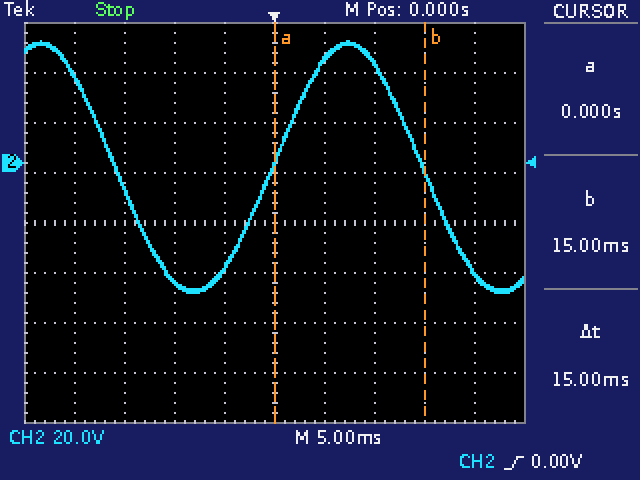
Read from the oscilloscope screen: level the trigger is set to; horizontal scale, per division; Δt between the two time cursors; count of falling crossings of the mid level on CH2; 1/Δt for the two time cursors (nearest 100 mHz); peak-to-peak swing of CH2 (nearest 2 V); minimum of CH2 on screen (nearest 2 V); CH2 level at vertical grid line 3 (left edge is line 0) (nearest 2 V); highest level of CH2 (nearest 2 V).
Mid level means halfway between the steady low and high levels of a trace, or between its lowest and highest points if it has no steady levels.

0.00 V
5 ms
15 ms
2
66.7 Hz
100 V
-52 V
-48 V
48 V
